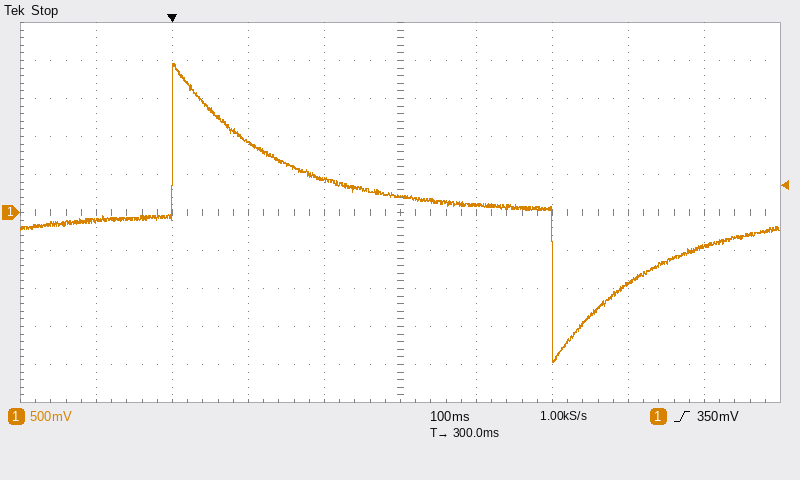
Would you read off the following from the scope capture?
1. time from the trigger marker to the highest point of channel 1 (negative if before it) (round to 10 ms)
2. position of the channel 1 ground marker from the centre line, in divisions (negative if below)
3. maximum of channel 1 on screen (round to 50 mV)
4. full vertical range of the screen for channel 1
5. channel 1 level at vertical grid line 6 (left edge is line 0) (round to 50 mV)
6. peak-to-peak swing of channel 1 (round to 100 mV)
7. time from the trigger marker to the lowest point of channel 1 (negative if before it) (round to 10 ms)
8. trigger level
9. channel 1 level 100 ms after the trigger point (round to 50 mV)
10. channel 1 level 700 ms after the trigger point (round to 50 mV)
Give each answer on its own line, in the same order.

0 ms
0.0 div
1.95 V
5 V
100 mV
3.90 V
+500 ms
350 mV
900 mV
-450 mV
